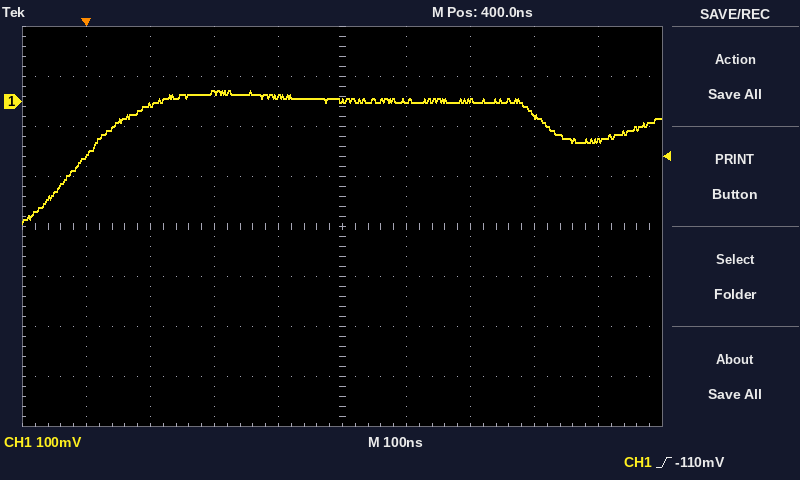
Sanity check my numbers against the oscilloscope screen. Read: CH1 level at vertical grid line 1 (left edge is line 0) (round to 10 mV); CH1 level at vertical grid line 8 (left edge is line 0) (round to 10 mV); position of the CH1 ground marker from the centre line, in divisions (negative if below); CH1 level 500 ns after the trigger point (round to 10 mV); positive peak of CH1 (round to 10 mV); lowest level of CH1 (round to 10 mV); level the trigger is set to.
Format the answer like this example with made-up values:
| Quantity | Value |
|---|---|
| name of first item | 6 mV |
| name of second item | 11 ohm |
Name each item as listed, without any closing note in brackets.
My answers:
| Quantity | Value |
|---|---|
| CH1 level at vertical grid line 1 (left edge is line 0) | -110 mV |
| CH1 level at vertical grid line 8 (left edge is line 0) | -30 mV |
| position of the CH1 ground marker from the centre line, in divisions | +2.5 div |
| CH1 level 500 ns after the trigger point | 0 mV |
| positive peak of CH1 | 20 mV |
| lowest level of CH1 | -240 mV |
| level the trigger is set to | -110 mV |
